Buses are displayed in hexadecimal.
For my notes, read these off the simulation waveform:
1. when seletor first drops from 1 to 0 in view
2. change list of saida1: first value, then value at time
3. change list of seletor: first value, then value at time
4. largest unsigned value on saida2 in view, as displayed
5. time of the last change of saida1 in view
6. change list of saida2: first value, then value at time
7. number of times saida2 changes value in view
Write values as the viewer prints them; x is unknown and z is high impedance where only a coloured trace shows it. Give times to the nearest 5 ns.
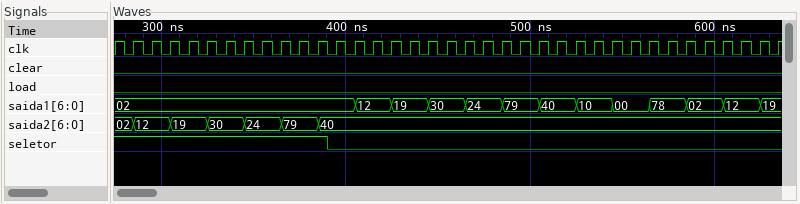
390 ns
02, 12 at 405 ns, 19 at 425 ns, 30 at 445 ns, 24 at 465 ns, 79 at 485 ns, 40 at 505 ns, 10 at 525 ns, 00 at 545 ns, 78 at 565 ns, 02 at 585 ns, 12 at 605 ns, 19 at 625 ns
1, 0 at 390 ns
79
625 ns
02, 12 at 285 ns, 19 at 305 ns, 30 at 325 ns, 24 at 345 ns, 79 at 365 ns, 40 at 385 ns
6
